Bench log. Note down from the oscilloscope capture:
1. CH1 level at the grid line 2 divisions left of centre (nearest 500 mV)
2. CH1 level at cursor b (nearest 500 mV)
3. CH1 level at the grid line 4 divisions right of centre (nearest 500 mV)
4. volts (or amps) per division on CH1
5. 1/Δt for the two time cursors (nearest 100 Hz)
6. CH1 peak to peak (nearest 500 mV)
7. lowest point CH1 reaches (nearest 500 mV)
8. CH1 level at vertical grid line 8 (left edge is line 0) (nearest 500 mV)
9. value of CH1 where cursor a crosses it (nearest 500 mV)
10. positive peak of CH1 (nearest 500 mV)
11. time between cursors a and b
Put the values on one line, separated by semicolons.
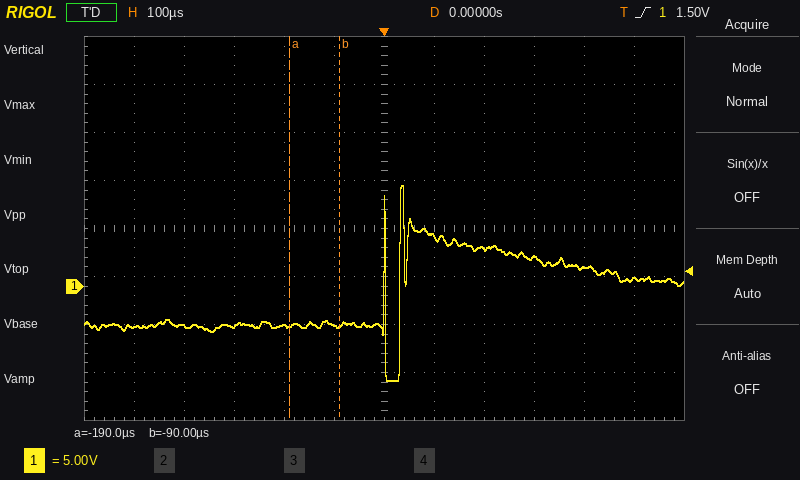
-4.0 V; -4.0 V; 2.0 V; 5 V; 10.0 kHz; 20.5 V; -10.0 V; 4.0 V; -4.0 V; 10.5 V; 100 µs
